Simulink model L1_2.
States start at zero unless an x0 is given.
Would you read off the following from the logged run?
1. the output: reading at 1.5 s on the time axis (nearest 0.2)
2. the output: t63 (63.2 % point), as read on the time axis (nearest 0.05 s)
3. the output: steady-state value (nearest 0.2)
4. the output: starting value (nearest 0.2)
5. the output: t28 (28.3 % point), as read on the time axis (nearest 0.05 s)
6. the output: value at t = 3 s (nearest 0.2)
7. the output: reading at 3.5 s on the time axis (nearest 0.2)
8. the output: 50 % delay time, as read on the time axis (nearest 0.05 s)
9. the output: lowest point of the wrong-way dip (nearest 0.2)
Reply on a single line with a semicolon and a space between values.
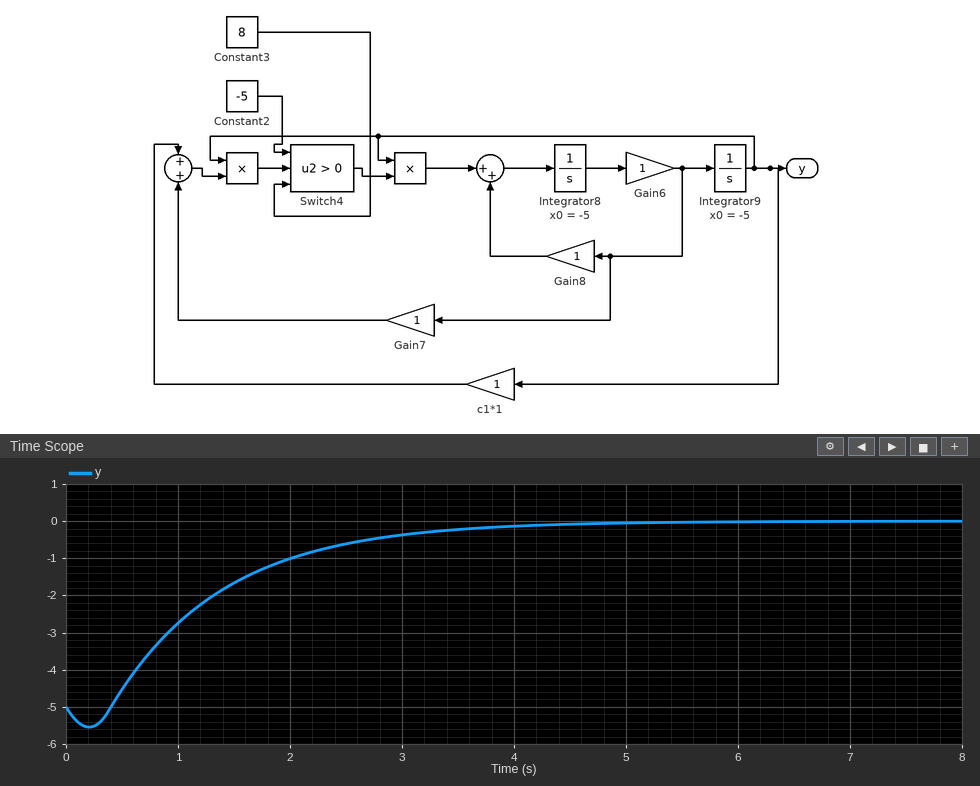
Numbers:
-1.6; 1.40 s; 0.0; -5.0; 0.75 s; -0.4; -0.2; 1.10 s; -5.6
